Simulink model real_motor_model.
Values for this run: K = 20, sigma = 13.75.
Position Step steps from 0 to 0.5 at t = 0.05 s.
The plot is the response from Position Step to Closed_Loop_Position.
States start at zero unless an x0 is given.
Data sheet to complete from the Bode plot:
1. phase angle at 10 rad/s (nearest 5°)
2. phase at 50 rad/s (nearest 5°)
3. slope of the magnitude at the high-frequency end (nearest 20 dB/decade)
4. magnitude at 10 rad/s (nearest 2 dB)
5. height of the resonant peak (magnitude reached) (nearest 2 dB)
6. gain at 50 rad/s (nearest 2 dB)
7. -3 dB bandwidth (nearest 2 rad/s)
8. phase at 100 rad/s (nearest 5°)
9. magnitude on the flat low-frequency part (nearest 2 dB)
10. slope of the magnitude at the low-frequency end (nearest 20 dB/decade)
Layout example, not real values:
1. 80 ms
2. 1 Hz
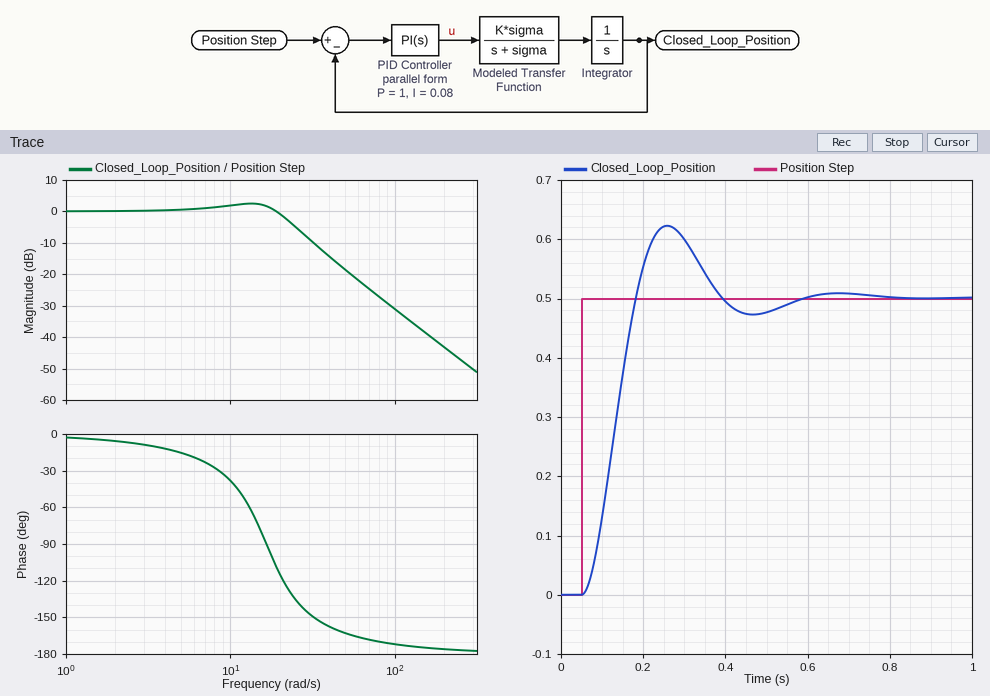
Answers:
1. -40°
2. -165°
3. -40 dB/decade
4. 2 dB
5. 2 dB
6. -18 dB
7. 22 rad/s
8. -170°
9. 0 dB
10. 0 dB/decade
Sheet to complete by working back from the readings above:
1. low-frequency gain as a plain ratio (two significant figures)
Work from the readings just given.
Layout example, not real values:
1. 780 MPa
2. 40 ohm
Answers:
1. 1.0
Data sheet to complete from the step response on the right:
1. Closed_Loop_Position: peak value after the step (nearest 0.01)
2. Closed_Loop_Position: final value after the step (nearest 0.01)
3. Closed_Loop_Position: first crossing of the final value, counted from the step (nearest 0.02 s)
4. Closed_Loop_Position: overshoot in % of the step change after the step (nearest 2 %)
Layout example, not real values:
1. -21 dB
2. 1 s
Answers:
1. 0.62
2. 0.50
3. 0.14 s
4. 24 %
